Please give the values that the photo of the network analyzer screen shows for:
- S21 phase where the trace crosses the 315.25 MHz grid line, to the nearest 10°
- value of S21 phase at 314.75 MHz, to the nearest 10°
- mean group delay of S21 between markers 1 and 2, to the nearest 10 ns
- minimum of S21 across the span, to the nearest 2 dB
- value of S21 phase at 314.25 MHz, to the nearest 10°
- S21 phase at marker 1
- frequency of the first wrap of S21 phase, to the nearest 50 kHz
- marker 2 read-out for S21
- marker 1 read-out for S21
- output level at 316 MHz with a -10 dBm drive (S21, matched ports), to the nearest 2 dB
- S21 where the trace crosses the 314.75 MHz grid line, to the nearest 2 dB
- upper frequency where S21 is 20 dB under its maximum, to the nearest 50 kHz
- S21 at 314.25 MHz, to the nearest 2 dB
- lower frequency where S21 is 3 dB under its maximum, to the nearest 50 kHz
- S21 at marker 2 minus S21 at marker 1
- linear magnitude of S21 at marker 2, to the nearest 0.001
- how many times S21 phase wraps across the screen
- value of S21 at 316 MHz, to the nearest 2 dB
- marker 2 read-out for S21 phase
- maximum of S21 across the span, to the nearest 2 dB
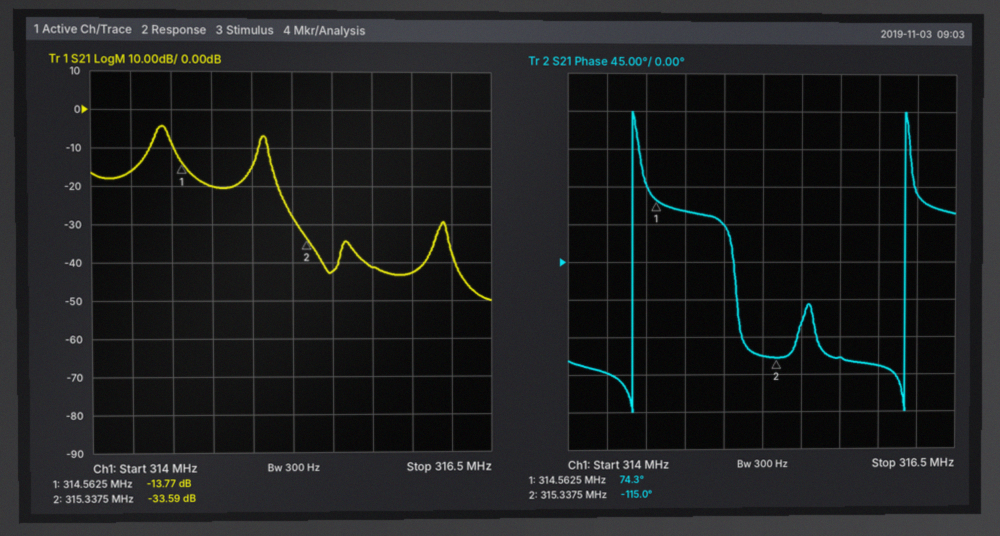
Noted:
-110°
60°
680 ns
-50 dB
-130°
74.3°
314.40 MHz
-33.59 dB
-13.77 dB
-52 dBm
-20 dB
315.20 MHz
-16 dB
314.40 MHz
-19.82 dB
0.021
2
-42 dB
-115.0°
-4 dB
